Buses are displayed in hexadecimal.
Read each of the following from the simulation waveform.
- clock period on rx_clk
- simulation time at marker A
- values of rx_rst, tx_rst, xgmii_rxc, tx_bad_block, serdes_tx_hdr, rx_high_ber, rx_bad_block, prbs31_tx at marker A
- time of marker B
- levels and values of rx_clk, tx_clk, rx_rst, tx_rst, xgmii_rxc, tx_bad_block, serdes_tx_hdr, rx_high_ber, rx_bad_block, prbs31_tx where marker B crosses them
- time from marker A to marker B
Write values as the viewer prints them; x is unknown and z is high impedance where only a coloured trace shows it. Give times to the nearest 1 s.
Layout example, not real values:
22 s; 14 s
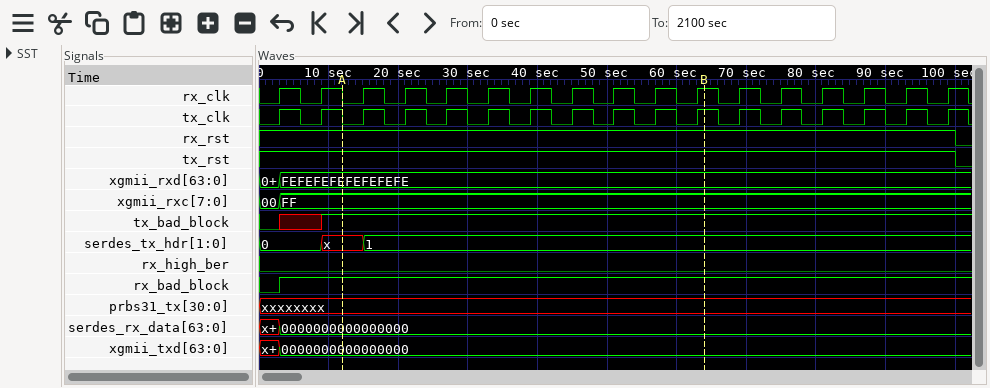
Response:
6 s; 12 s; rx_rst=1, tx_rst=1, xgmii_rxc=FF, tx_bad_block=1, serdes_tx_hdr=x, rx_high_ber=0, rx_bad_block=1, prbs31_tx=xxxxxxxx; 64 s; rx_clk=1, tx_clk=1, rx_rst=1, tx_rst=1, xgmii_rxc=FF, tx_bad_block=1, serdes_tx_hdr=1, rx_high_ber=0, rx_bad_block=1, prbs31_tx=xxxxxxxx; 52 s
